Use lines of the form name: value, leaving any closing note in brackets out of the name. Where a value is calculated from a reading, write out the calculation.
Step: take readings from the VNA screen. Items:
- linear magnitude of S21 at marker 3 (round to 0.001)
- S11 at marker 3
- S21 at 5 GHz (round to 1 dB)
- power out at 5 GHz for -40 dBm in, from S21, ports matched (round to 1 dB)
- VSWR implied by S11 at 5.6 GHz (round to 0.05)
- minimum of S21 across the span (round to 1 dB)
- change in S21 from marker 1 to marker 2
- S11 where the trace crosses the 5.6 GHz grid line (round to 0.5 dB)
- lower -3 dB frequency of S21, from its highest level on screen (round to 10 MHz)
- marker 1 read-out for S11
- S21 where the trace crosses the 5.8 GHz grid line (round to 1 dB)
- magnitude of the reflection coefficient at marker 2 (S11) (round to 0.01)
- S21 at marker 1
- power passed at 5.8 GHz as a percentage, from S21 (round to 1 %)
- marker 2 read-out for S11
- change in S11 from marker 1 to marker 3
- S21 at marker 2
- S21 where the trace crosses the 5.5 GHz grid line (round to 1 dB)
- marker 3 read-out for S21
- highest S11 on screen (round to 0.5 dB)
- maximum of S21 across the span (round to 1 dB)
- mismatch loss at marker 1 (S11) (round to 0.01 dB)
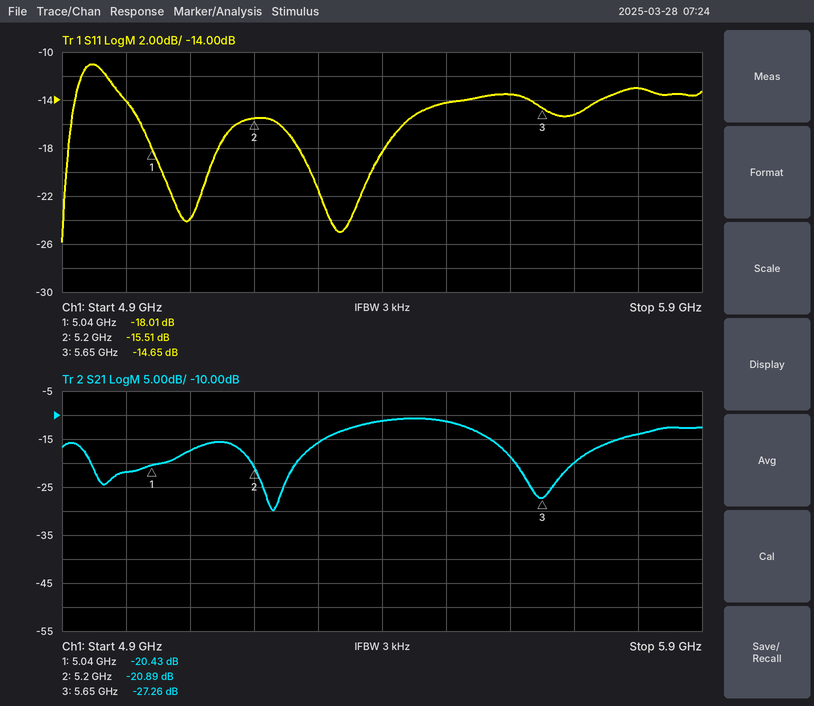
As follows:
linear magnitude of S21 at marker 3: 10^(-27.26/20) ≈ 0.043
S11 at marker 3: -14.65 dB
S21 at 5 GHz: -22 dB
power out at 5 GHz for -40 dBm in, from S21, ports matched: -40 dBm + (-22 dB) = -62 dBm
VSWR implied by S11 at 5.6 GHz: |Γ| = 10^(-13.5/20) = 0.2113; VSWR = (1 + 0.2113)/(1 − 0.2113) ≈ 1.54, so 1.55 to the nearest 0.05
minimum of S21 across the span: -30 dB
change in S21 from marker 1 to marker 2: -20.89 − (-20.43) = -0.46 dB
S11 where the trace crosses the 5.6 GHz grid line: -13.5 dB
lower -3 dB frequency of S21, from its highest level on screen: 5.33 GHz
marker 1 read-out for S11: -18.01 dB
S21 where the trace crosses the 5.8 GHz grid line: -14 dB
magnitude of the reflection coefficient at marker 2 (S11): 10^(-15.51/20) ≈ 0.17
S21 at marker 1: -20.43 dB
power passed at 5.8 GHz as a percentage, from S21: 10^(-14/10) ≈ 4 %
marker 2 read-out for S11: -15.51 dB
change in S11 from marker 1 to marker 3: -14.65 − (-18.01) = 3.36 dB
S21 at marker 2: -20.89 dB
S21 where the trace crosses the 5.5 GHz grid line: -11 dB
marker 3 read-out for S21: -27.26 dB
highest S11 on screen: -11.0 dB
maximum of S21 across the span: -11 dB
mismatch loss at marker 1 (S11): −10 log10(1 − 10^(-18.01/10)) ≈ 0.07 dB
